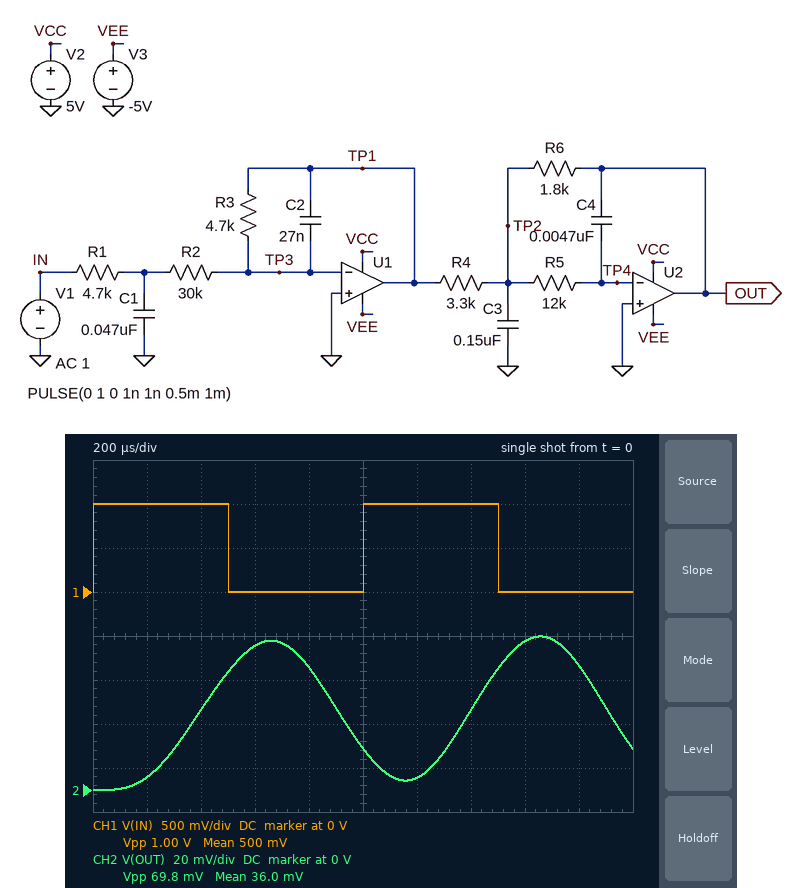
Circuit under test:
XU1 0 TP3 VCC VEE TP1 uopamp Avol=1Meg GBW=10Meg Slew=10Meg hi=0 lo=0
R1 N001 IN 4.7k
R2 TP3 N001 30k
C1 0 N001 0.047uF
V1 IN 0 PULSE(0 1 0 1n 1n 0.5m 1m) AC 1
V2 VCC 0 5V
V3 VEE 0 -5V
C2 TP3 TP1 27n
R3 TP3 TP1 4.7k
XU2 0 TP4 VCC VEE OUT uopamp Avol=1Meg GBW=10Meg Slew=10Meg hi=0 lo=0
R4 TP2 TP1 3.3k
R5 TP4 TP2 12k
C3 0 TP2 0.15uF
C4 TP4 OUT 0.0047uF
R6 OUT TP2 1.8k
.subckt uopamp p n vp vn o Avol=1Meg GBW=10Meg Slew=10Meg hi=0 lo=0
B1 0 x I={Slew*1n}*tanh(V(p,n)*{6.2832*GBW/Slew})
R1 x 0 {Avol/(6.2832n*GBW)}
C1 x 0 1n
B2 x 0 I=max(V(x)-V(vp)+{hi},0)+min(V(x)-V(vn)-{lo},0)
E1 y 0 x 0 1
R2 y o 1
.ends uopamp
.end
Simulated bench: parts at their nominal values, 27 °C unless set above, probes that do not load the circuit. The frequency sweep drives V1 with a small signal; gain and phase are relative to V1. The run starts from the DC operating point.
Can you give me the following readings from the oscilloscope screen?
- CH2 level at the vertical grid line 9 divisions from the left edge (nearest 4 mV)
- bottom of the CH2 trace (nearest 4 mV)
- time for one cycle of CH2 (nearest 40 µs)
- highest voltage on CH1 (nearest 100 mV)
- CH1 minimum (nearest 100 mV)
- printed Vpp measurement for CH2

56 mV
0 V
1.00 ms
1.0 V
0 V
69.8 mV
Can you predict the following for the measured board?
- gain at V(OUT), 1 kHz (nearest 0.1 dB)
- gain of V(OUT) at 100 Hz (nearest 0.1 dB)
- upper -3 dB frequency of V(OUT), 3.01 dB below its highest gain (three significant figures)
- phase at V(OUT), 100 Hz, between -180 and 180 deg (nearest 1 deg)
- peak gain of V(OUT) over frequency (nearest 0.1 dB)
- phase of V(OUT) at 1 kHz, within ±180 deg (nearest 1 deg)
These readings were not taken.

-25.8 dB
-22.7 dB
974 Hz
-15 deg
-22.6 dB
-145 deg
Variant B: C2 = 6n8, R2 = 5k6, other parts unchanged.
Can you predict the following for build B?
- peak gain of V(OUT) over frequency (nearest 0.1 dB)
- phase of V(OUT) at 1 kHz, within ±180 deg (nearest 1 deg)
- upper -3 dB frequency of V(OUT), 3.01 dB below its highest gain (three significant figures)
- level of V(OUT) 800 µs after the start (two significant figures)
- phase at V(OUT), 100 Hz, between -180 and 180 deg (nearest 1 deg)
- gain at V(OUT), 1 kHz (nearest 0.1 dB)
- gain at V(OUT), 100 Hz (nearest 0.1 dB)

-11.3 dB
-105 deg
1.40 kHz
110 mV
-9 deg
-11.4 dB
-12.1 dB
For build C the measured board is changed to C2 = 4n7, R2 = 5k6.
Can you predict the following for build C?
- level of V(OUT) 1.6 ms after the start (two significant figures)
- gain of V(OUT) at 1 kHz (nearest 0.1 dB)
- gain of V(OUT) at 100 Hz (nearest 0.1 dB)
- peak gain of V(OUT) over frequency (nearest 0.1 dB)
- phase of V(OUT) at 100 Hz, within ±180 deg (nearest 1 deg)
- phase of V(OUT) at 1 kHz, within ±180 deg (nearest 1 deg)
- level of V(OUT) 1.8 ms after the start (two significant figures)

290 mV
-11.3 dB
-12.1 dB
-11.2 dB
-9 deg
-101 deg
100 mV
